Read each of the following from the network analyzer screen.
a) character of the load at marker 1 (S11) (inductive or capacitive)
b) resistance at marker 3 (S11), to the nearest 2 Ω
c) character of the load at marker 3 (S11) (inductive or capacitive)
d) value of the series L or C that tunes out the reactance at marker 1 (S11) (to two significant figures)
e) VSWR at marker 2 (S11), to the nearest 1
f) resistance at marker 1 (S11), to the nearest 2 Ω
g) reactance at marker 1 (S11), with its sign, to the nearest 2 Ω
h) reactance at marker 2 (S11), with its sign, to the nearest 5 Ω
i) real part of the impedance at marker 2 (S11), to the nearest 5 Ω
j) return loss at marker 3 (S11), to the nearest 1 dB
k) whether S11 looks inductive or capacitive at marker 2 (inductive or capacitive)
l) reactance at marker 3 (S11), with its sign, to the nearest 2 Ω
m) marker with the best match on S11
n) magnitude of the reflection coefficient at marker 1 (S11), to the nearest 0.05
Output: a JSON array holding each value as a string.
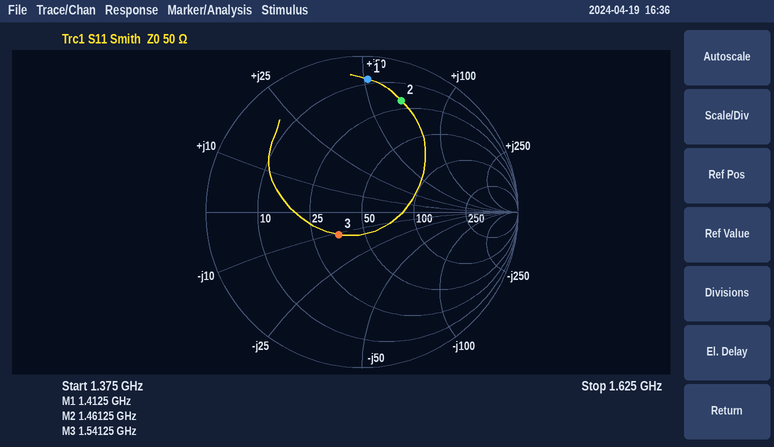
["inductive", "36 Ω", "capacitive", "2.2 pF", "7", "8 Ω", "+52 Ω", "+65 Ω", "20 Ω", "14 dB", "inductive", "-10 Ω", "marker 3", "0.85"]
